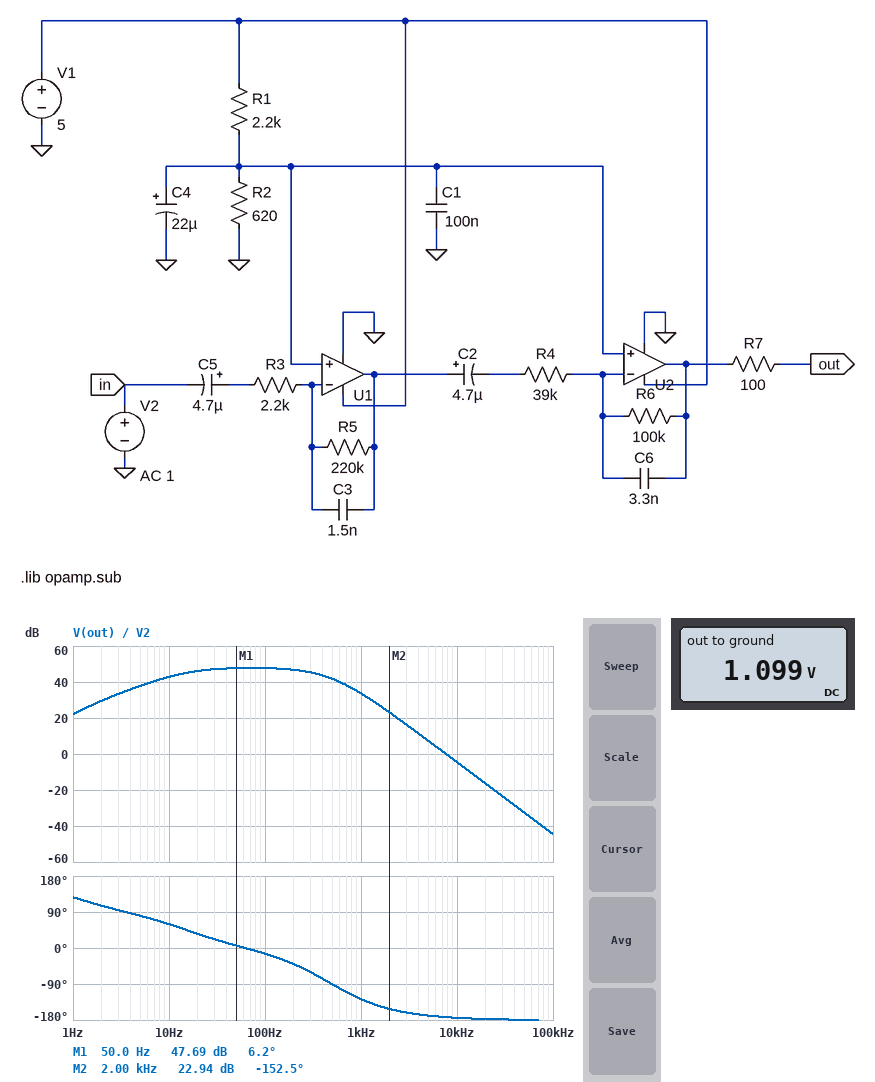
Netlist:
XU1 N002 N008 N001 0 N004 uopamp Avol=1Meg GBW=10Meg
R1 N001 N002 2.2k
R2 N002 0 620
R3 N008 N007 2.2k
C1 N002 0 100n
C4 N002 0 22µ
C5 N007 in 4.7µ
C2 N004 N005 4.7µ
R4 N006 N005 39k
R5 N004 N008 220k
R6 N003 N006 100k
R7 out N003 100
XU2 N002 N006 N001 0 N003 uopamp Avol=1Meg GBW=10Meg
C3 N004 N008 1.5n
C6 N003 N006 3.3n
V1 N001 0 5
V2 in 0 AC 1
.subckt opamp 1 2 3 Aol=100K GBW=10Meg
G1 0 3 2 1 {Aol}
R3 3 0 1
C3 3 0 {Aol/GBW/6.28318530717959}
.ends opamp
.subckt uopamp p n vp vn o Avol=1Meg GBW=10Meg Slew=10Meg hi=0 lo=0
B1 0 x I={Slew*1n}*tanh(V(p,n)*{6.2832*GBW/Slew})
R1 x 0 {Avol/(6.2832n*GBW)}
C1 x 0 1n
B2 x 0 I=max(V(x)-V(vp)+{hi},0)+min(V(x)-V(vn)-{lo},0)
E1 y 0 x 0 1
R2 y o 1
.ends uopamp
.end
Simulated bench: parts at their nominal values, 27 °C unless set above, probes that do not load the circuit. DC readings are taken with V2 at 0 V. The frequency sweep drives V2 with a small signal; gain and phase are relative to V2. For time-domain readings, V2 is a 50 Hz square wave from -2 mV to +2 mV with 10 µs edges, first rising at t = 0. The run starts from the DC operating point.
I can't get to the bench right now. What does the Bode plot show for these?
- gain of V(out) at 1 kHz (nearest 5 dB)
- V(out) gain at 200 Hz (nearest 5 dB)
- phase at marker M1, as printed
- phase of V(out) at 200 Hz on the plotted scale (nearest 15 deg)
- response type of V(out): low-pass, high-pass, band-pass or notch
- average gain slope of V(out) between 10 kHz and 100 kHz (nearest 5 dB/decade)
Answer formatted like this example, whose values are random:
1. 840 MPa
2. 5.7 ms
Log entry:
1. 35 dB
2. 45 dB
3. 6.2 deg
4. -45 deg
5. band-pass
6. -40 dB/decade
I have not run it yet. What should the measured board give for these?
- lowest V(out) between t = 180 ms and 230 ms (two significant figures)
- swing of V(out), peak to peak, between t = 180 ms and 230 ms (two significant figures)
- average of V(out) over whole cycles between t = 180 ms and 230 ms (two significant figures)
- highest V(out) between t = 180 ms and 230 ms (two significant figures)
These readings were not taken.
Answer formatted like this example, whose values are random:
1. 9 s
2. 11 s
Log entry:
1. 440 mV
2. 1.3 V
3. 1.1 V
4. 1.7 V
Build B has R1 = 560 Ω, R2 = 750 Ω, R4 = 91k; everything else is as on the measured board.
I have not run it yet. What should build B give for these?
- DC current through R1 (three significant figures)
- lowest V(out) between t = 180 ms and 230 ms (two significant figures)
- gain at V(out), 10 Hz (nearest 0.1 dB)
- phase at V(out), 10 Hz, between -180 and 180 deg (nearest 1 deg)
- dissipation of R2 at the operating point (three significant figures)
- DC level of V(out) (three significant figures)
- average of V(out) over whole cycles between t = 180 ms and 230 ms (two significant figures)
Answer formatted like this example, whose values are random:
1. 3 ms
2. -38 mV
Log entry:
1. 3.82 mA
2. 2.6 V
3. 35.5 dB
4. 57 deg
5. 10.9 mW
6. 2.86 V
7. 2.9 V
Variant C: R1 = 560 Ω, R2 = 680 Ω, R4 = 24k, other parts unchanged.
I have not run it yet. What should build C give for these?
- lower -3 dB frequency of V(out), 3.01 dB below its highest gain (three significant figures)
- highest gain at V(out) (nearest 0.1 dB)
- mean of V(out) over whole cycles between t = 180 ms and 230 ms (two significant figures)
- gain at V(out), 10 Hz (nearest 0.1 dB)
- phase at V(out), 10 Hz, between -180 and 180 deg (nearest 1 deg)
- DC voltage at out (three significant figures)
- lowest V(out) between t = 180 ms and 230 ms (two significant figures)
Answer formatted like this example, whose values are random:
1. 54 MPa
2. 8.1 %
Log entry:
1. 14.3 Hz
2. 52.0 dB
3. 2.7 V
4. 47.0 dB
5. 63 deg
6. 2.74 V
7. 1.7 V
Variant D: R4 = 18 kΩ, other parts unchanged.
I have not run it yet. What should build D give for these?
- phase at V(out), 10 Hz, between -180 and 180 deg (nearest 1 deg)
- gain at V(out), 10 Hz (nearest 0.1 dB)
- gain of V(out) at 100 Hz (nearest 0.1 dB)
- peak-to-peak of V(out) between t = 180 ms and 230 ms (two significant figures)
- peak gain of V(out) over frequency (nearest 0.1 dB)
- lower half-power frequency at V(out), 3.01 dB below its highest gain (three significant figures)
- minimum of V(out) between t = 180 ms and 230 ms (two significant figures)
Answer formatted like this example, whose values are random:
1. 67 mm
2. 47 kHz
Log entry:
1. 65 deg
2. 49.5 dB
3. 54.4 dB
4. 2.5 V
5. 54.5 dB
6. 14.4 Hz
7. -3.7 mV
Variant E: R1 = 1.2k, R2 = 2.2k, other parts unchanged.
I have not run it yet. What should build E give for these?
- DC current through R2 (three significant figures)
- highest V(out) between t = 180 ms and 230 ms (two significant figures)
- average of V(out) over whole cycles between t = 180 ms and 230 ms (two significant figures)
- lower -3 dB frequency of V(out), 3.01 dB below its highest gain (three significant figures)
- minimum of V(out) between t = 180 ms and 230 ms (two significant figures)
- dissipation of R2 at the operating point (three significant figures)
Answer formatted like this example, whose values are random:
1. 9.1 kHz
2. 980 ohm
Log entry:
1. 1.47 mA
2. 3.9 V
3. 3.2 V
4. 14.2 Hz
5. 2.6 V
6. 4.76 mW
